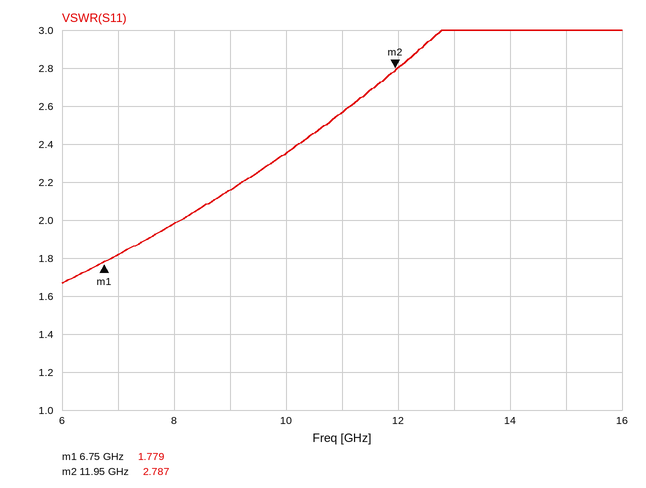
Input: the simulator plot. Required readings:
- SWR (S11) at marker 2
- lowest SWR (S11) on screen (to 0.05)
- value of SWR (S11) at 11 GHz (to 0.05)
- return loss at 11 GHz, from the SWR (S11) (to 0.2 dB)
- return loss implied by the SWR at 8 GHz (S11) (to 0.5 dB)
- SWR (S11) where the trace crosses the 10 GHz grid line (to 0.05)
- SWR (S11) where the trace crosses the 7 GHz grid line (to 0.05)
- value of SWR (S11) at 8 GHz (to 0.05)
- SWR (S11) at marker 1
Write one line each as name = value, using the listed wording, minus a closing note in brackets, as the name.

SWR (S11) at marker 2 = 2.787
lowest SWR (S11) on screen = 1.65
value of SWR (S11) at 11 GHz = 2.55
return loss at 11 GHz, from the SWR (S11) = 7.2 dB
return loss implied by the SWR at 8 GHz (S11) = 9.5 dB
SWR (S11) where the trace crosses the 10 GHz grid line = 2.35
SWR (S11) where the trace crosses the 7 GHz grid line = 1.80
value of SWR (S11) at 8 GHz = 2.00
SWR (S11) at marker 1 = 1.779
